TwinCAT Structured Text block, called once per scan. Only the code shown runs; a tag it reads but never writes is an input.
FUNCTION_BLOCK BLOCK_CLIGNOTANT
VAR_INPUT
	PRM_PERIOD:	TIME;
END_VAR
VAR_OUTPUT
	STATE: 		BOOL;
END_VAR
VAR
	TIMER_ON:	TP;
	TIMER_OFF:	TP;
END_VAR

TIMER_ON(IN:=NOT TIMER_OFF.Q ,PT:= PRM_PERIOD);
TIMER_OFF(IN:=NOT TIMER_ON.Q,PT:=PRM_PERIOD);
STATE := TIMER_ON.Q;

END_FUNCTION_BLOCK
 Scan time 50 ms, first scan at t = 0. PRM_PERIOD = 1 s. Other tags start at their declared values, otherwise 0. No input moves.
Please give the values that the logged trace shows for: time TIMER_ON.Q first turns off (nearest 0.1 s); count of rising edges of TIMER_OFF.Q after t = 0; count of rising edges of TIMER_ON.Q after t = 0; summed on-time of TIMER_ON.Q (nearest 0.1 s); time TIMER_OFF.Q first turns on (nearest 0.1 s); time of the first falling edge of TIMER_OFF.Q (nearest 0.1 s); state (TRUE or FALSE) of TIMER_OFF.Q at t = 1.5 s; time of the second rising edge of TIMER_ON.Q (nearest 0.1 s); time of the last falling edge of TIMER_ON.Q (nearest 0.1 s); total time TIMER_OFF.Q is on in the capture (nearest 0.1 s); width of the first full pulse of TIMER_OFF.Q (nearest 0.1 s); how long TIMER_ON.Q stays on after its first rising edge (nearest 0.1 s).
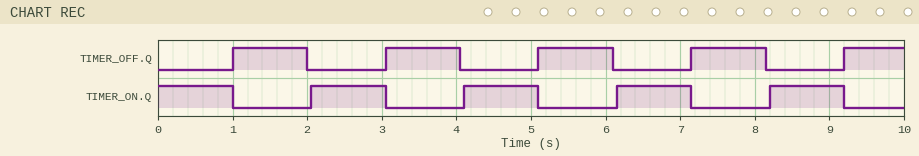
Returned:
1.0 s
5
4
5.0 s
1.0 s
2.0 s
TRUE
4.1 s
9.2 s
4.8 s
1.0 s
1.0 s
